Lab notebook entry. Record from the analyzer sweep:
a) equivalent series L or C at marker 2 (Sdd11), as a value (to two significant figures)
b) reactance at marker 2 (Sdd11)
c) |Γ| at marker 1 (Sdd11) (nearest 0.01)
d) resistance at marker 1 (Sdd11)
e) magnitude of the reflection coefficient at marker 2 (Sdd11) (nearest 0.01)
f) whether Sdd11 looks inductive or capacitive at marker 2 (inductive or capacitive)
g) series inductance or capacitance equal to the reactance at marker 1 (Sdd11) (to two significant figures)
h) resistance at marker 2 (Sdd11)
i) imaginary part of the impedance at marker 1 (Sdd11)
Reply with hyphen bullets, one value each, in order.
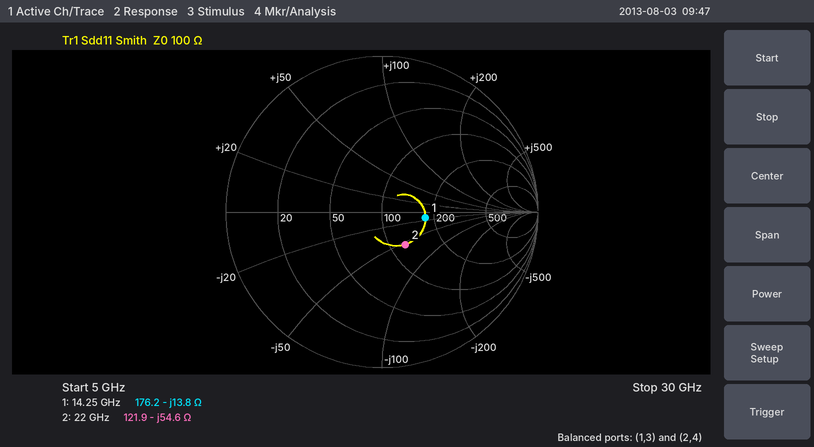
- 130 fF
- -54.6 Ω
- 0.28
- 176.2 Ω
- 0.26
- capacitive
- 810 fF
- 121.9 Ω
- -13.8 Ω
